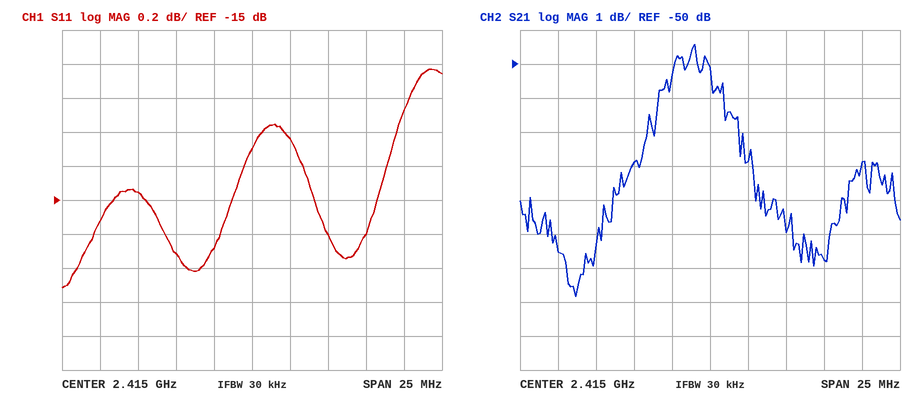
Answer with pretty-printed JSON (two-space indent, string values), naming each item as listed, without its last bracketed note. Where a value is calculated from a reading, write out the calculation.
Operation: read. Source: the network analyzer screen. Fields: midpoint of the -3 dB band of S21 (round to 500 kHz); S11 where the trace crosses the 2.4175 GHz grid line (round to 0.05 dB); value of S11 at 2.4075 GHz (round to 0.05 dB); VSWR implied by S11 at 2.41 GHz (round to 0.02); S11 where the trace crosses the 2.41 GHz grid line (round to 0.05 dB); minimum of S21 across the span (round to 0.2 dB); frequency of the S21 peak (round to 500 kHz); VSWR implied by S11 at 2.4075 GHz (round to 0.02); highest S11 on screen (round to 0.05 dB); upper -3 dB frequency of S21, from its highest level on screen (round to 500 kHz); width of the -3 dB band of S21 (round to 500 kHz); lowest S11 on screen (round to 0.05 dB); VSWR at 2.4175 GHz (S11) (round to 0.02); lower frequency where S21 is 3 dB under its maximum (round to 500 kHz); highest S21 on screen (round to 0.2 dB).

{
  "midpoint of the -3 dB band of S21": "2.4140 GHz",
  "S11 where the trace crosses the 2.4175 GHz grid line": "-14.65 dB",
  "value of S11 at 2.4075 GHz": "-14.95 dB",
  "VSWR implied by S11 at 2.41 GHz": "|Γ| = 10^(-15.3/20) = 0.1718; VSWR = (1 + 0.1718)/(1 − 0.1718) ≈ 1.41, so 1.42 to the nearest 0.02",
  "S11 where the trace crosses the 2.41 GHz grid line": "-15.30 dB",
  "minimum of S21 across the span": "-56.8 dB",
  "frequency of the S21 peak": "2.4140 GHz",
  "VSWR implied by S11 at 2.4075 GHz": "|Γ| = 10^(-14.95/20) = 0.1789; VSWR = (1 + 0.1789)/(1 − 0.1789) ≈ 1.44",
  "highest S11 on screen": "-14.25 dB",
  "upper -3 dB frequency of S21, from its highest level on screen": "2.4170 GHz",
  "width of the -3 dB band of S21": "2.4170 GHz − 2.4105 GHz = 6.5 MHz",
  "lowest S11 on screen": "-15.50 dB",
  "VSWR at 2.4175 GHz (S11)": "|Γ| = 10^(-14.65/20) = 0.1851; VSWR = (1 + 0.1851)/(1 − 0.1851) ≈ 1.45, so 1.46 to the nearest 0.02",
  "lower frequency where S21 is 3 dB under its maximum": "2.4105 GHz",
  "highest S21 on screen": "-49.4 dB"
}
